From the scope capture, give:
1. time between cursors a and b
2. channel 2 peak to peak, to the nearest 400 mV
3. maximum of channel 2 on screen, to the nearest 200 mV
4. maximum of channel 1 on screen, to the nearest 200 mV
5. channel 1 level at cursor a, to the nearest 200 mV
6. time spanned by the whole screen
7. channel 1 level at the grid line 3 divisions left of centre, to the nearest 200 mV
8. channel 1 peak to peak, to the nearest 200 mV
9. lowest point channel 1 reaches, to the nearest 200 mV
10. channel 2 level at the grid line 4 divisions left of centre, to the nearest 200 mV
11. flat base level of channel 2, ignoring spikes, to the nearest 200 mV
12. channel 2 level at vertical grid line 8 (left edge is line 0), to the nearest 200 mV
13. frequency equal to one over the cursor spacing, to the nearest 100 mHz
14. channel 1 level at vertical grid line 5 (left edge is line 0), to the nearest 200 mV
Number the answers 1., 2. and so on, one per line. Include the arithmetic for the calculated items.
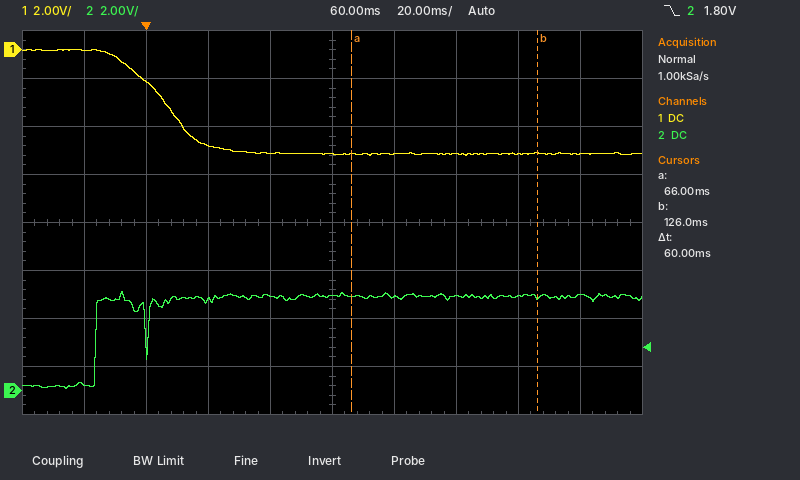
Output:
1. 60 ms
2. 4.0 V
3. 4.2 V
4. 0.0 V
5. -4.4 V
6. 200 ms
7. -1.4 V
8. 0.0 V − (-4.4 V) = 4.4 V
9. -4.4 V
10. 200 mV
11. 200 mV
12. 4.0 V
13. 1 / 60 ms ≈ 16.7 Hz
14. -4.4 V
